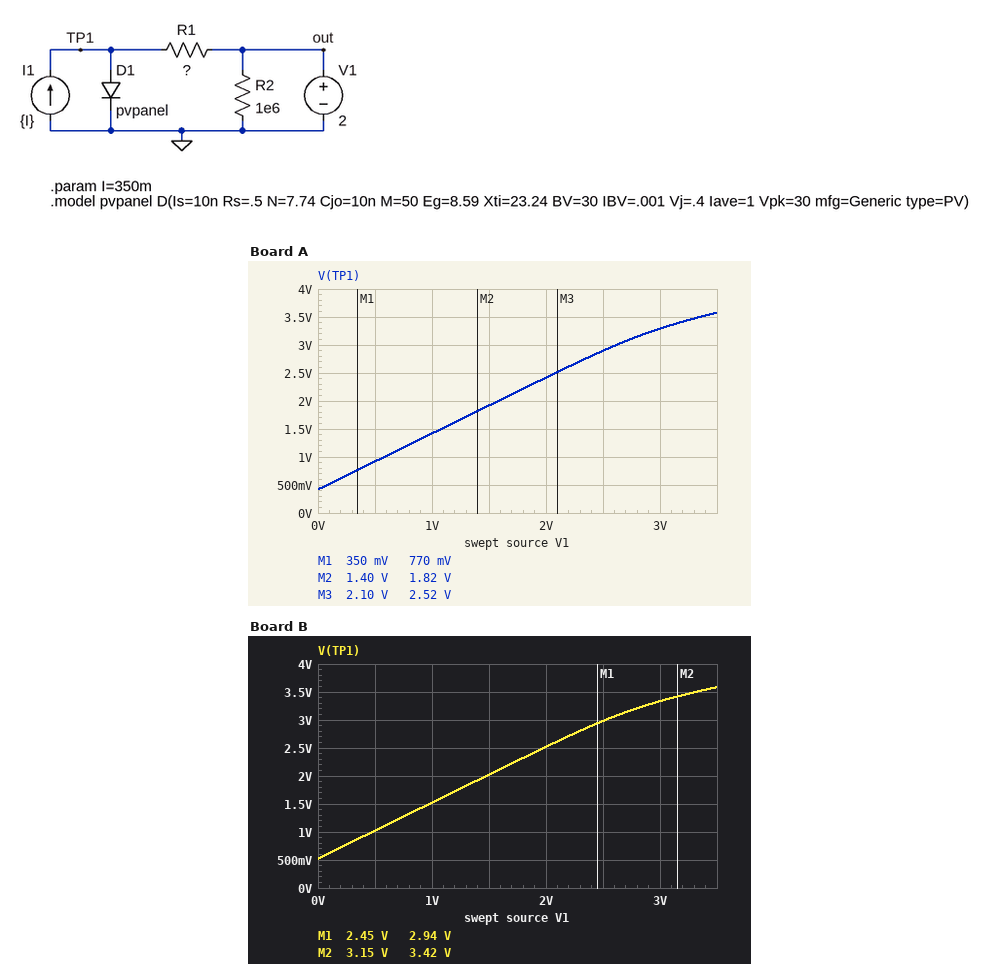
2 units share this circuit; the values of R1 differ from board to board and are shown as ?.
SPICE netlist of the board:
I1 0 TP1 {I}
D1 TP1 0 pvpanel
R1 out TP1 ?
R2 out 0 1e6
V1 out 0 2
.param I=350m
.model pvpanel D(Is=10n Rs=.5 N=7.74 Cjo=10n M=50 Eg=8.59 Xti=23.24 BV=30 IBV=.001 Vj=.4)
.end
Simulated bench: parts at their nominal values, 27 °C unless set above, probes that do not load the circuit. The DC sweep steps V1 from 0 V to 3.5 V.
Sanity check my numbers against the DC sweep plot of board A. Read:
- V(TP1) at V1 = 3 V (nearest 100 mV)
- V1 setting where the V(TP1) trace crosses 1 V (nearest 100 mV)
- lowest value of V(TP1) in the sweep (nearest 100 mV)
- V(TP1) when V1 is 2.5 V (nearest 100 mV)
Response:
3.3 V
600 mV
400 mV
2.9 V
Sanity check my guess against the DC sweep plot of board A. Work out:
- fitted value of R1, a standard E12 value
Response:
1.2 Ω
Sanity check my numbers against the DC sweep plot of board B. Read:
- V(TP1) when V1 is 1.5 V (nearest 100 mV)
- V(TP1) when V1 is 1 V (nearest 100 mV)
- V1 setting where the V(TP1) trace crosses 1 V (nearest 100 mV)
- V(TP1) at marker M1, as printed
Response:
2.0 V
1.5 V
500 mV
2.94 V
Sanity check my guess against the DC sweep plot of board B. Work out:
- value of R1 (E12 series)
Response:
1.5 Ω
